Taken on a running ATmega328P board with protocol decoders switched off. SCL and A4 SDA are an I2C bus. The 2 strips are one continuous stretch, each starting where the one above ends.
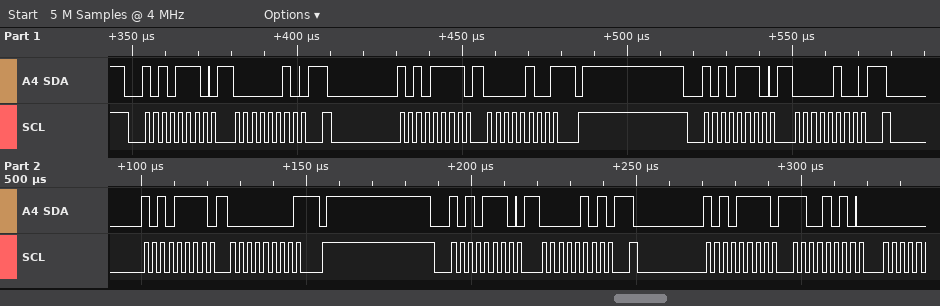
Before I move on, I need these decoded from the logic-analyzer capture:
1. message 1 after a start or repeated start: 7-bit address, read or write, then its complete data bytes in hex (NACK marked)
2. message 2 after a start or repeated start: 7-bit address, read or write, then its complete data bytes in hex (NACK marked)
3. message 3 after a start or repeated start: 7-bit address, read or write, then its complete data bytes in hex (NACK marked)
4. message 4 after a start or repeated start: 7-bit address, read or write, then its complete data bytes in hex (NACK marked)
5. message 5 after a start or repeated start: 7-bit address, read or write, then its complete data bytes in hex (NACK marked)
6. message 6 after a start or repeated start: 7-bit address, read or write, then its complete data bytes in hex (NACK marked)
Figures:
0x57 write: 02
0x57 read: 04 NACK
0x57 write: 04
0x57 read: 00 NACK
0x57 write: 05
0x57 read: CA
